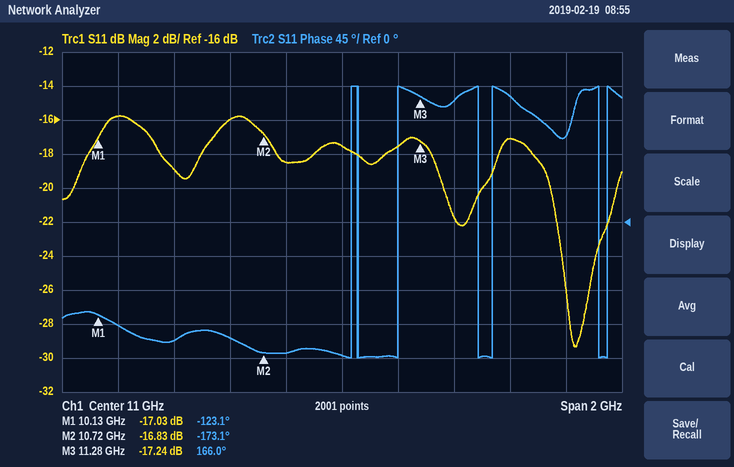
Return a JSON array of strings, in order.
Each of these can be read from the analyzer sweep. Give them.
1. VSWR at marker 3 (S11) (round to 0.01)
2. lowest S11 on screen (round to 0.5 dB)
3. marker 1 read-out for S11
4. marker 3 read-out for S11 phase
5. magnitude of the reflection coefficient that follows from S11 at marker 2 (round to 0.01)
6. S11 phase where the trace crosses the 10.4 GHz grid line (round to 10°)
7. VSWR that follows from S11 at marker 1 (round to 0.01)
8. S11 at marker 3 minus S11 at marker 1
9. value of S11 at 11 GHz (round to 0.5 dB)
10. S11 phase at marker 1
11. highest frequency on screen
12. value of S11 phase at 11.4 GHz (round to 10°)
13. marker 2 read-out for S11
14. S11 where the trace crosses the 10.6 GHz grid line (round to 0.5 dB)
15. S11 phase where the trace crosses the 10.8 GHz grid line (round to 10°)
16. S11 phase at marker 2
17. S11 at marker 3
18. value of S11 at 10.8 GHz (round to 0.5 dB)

["1.32", "-29.5 dB", "-17.03 dB", "166.0°", "0.14", "-160°", "1.33", "-0.21 dB", "-17.5 dB", "-123.1°", "12 GHz", "160°", "-16.83 dB", "-16.0 dB", "-170°", "-173.1°", "-17.24 dB", "-18.5 dB"]
